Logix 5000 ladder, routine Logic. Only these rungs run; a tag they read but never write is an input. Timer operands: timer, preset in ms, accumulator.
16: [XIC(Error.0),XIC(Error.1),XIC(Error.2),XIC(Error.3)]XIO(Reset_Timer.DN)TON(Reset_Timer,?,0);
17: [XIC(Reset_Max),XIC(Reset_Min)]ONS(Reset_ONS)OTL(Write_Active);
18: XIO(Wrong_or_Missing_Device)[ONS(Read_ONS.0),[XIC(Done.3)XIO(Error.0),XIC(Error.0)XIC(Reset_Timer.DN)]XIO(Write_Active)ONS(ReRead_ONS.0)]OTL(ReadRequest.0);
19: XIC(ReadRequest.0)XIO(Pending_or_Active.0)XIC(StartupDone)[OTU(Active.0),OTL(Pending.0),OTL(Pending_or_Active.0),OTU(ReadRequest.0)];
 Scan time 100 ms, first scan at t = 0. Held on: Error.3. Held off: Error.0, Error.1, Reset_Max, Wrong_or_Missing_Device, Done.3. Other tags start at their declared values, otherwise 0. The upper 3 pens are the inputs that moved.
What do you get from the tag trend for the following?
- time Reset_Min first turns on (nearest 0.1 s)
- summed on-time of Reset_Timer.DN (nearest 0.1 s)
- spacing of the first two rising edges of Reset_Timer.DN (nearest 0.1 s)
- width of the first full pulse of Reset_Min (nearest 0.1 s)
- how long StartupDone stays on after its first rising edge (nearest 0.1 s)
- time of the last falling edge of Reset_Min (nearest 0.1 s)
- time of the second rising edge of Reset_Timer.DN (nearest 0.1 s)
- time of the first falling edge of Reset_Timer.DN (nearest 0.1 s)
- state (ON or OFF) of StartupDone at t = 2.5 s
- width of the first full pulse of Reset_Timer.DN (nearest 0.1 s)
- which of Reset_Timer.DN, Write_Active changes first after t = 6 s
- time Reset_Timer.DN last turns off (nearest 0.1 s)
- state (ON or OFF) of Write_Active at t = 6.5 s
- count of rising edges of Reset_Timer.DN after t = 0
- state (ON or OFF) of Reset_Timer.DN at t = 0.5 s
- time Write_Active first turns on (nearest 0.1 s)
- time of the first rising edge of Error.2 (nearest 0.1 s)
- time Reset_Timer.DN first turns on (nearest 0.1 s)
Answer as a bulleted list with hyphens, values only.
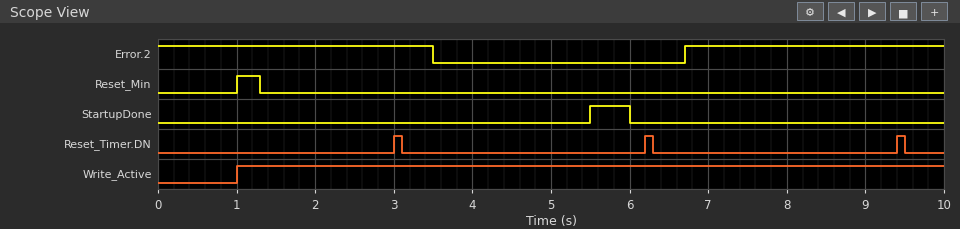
- 1.0 s
- 0.3 s
- 3.2 s
- 0.3 s
- 0.5 s
- 1.3 s
- 6.2 s
- 3.1 s
- OFF
- 0.1 s
- Reset_Timer.DN
- 9.5 s
- ON
- 3
- OFF
- 1.0 s
- 6.7 s
- 3.0 s
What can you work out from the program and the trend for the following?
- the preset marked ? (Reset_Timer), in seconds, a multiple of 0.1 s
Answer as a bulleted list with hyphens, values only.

- 3.0 s
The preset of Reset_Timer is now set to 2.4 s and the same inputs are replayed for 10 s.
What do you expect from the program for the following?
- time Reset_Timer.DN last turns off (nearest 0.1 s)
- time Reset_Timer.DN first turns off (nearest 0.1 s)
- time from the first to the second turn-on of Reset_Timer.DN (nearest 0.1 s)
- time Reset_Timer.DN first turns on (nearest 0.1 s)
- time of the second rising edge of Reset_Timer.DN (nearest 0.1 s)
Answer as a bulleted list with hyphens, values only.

- 7.7 s
- 2.5 s
- 2.6 s
- 2.4 s
- 5.0 s
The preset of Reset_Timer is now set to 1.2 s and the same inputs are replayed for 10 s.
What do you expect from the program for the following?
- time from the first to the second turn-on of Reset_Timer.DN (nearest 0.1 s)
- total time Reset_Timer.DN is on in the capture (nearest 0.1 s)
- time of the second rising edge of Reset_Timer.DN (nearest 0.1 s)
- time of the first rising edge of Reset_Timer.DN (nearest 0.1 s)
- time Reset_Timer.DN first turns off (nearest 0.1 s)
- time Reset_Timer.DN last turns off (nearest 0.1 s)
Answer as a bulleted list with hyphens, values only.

- 1.4 s
- 0.7 s
- 2.6 s
- 1.2 s
- 1.3 s
- 9.7 s
